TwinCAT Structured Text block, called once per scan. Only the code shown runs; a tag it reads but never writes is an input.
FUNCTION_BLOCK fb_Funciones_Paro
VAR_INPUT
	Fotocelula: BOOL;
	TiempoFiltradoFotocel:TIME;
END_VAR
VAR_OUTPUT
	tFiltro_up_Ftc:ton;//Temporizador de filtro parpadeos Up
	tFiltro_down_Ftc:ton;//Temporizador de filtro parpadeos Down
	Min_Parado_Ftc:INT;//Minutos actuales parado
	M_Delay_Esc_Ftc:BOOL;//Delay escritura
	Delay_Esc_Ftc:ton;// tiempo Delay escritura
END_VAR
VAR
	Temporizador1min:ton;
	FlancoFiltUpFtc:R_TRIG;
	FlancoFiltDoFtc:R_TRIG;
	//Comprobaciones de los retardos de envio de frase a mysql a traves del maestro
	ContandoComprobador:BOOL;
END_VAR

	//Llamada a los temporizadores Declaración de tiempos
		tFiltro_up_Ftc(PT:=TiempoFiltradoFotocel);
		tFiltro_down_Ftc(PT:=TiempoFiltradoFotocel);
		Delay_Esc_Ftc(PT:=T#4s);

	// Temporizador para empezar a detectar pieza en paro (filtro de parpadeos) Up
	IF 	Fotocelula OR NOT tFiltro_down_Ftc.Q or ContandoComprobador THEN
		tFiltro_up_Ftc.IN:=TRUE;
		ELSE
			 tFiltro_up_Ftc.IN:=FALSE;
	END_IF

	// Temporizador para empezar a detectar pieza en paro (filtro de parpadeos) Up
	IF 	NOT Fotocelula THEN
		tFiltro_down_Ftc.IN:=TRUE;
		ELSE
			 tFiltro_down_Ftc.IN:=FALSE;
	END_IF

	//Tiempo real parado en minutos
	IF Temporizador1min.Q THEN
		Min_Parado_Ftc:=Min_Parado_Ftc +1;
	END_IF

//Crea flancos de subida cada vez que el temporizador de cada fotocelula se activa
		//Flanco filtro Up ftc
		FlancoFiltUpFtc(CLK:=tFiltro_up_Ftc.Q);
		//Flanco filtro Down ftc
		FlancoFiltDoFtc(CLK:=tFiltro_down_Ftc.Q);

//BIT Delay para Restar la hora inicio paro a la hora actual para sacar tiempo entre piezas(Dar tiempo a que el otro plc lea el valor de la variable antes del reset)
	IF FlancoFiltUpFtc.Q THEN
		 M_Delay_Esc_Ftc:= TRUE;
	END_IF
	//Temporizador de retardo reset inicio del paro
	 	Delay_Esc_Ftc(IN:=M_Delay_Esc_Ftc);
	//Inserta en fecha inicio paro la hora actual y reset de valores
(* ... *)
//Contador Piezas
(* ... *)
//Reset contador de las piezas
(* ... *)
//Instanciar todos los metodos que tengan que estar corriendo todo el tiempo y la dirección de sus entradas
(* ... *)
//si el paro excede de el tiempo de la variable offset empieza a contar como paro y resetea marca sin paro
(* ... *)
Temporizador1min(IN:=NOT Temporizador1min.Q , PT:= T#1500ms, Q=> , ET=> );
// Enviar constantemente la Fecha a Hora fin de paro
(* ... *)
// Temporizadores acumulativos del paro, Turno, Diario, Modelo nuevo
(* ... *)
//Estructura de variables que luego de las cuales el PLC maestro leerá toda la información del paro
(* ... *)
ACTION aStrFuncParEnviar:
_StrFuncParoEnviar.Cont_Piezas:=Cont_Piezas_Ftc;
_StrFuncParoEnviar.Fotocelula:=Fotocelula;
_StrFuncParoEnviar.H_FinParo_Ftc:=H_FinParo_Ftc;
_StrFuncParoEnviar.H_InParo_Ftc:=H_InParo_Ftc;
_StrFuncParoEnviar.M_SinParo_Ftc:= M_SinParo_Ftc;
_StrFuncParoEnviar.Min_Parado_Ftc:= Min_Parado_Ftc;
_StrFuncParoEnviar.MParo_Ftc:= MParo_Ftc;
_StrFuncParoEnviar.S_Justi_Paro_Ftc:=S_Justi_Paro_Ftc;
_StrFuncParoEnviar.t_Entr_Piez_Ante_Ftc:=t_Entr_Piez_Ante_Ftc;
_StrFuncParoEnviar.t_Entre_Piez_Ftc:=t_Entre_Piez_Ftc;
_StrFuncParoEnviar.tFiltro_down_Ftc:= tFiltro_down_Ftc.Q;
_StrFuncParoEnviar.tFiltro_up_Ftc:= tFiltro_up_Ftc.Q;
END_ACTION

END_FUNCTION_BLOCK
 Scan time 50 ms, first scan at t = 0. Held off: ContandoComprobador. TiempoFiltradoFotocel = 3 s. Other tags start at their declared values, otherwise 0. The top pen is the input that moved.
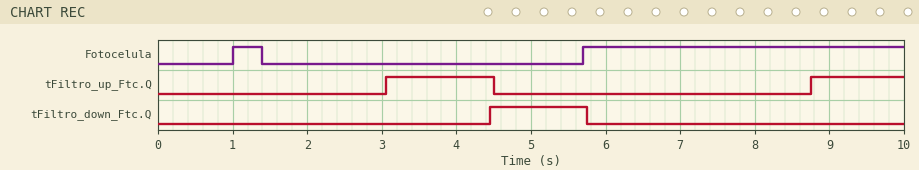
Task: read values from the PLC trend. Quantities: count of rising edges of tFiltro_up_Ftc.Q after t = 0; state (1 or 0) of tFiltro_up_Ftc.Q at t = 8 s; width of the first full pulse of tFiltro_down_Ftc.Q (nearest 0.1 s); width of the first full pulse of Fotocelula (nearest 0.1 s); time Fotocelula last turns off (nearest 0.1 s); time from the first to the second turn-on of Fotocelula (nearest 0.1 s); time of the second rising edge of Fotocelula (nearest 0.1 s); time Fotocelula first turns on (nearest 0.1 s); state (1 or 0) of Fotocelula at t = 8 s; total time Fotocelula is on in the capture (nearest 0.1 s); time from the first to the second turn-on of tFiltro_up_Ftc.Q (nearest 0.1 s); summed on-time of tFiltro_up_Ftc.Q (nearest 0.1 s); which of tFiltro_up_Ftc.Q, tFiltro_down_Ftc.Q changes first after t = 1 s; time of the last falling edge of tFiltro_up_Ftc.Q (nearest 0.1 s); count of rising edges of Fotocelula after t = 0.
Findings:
2
0
1.3 s
0.4 s
1.4 s
4.7 s
5.7 s
1.0 s
1
4.7 s
5.7 s
2.7 s
tFiltro_up_Ftc.Q
4.5 s
2
